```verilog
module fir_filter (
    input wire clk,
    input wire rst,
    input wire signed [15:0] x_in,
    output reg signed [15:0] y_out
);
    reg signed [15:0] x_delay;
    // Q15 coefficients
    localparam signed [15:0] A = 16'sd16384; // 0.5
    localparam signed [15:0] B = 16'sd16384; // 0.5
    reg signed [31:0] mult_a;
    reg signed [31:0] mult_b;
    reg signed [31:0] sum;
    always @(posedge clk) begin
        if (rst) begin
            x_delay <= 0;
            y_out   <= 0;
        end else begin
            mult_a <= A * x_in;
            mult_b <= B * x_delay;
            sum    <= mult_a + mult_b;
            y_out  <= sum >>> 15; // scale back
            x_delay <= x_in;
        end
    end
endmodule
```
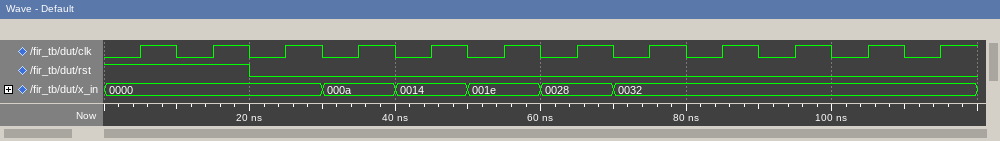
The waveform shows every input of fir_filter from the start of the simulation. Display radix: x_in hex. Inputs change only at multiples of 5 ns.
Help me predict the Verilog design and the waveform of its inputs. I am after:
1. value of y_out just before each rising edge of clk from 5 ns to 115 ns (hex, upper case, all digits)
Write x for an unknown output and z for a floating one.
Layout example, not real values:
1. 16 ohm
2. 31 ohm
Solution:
1. x, 0000, 0000, x, x, 0000, 0005, 000F, 0019, 0023, 002D, 0032
